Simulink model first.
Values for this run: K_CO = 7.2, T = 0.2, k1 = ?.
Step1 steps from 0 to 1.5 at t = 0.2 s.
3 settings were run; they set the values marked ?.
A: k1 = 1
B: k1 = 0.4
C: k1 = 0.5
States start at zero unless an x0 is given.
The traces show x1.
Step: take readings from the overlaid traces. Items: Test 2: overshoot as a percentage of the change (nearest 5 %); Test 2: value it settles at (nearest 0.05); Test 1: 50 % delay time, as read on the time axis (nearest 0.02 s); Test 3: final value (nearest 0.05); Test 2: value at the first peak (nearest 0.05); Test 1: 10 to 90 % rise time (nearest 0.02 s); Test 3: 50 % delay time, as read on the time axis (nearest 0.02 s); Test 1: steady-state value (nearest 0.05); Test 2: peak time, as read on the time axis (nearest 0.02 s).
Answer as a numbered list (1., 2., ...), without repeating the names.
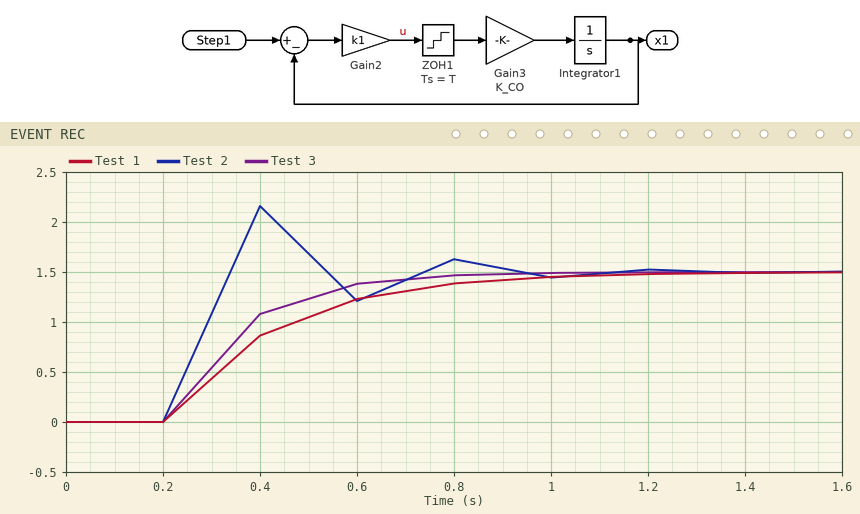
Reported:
1. 45 %
2. 1.50
3. 0.38 s
4. 1.50
5. 2.15
6. 0.52 s
7. 0.34 s
8. 1.50
9. 0.40 s
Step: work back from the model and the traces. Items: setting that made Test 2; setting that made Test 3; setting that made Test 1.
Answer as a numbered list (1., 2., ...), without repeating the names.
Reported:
1. A
2. C
3. B
